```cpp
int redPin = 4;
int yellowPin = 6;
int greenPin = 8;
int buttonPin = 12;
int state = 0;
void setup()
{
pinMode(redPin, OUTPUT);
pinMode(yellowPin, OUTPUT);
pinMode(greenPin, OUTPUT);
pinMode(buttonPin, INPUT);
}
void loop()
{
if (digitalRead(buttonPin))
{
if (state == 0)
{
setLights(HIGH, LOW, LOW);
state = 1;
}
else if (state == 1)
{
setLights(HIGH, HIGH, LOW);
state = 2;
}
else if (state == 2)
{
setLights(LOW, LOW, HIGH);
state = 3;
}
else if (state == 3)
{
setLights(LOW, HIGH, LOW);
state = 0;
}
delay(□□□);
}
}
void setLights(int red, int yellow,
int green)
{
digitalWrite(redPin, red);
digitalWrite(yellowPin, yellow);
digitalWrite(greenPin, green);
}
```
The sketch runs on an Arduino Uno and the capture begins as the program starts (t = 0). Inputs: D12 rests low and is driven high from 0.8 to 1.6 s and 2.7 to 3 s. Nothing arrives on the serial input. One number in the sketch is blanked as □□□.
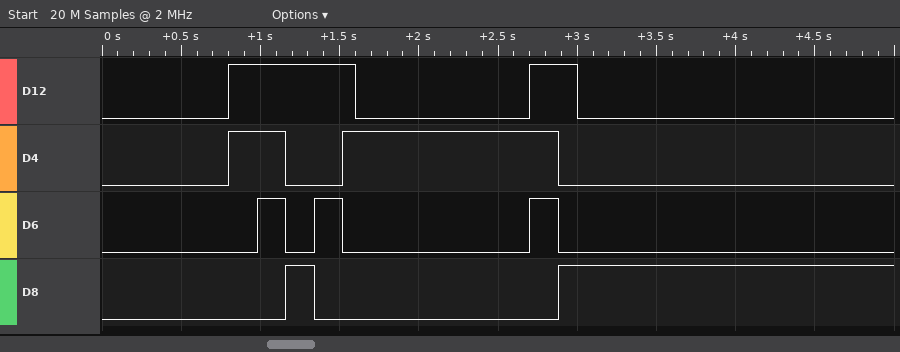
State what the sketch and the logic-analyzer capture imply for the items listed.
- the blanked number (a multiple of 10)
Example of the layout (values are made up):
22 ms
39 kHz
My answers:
180
